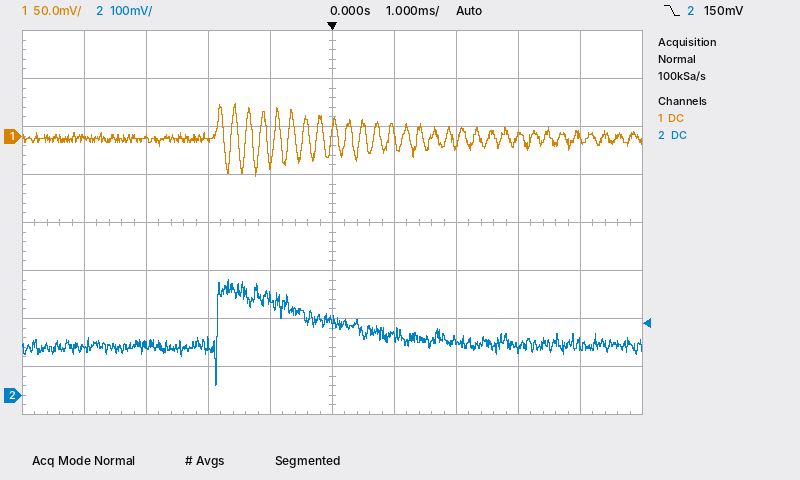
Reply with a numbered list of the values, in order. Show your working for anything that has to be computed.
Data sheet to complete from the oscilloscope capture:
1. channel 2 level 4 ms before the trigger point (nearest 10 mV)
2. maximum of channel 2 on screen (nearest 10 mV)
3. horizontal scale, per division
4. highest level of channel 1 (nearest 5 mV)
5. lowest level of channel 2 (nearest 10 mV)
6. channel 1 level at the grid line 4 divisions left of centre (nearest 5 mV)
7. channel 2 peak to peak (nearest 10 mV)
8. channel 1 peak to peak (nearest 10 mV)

1. 100 mV
2. 240 mV
3. 1 ms
4. 35 mV
5. 20 mV
6. 0 mV
7. 240 mV − (20 mV) = 220 mV
8. 80 mV
